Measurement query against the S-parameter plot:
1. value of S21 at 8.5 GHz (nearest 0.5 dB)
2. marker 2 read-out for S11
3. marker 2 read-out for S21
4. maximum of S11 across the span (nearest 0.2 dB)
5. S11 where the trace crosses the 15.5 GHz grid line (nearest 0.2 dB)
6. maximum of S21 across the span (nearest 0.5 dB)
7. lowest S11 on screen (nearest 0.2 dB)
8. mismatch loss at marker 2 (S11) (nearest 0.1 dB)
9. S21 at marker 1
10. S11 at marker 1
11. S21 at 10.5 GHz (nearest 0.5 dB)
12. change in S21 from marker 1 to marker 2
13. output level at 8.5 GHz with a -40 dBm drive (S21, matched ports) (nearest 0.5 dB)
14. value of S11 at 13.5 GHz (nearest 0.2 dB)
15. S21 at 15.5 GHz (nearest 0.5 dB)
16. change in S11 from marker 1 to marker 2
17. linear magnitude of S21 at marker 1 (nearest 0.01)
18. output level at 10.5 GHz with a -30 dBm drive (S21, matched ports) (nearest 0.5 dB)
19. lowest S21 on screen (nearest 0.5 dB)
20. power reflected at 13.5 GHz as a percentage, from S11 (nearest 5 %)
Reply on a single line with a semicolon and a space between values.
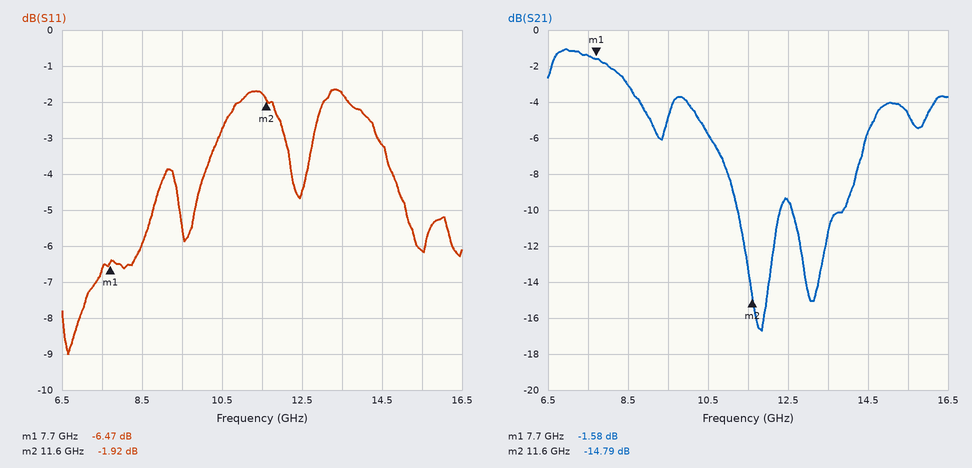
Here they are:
-3.0 dB; -1.92 dB; -14.79 dB; -1.6 dB; -6.2 dB; -1.0 dB; -9.0 dB; 4.5 dB; -1.58 dB; -6.47 dB; -6.0 dB; -13.21 dB; -43.0 dBm; -1.8 dB; -4.5 dB; 4.55 dB; 0.83; -36.0 dBm; -16.5 dB; 65 %
